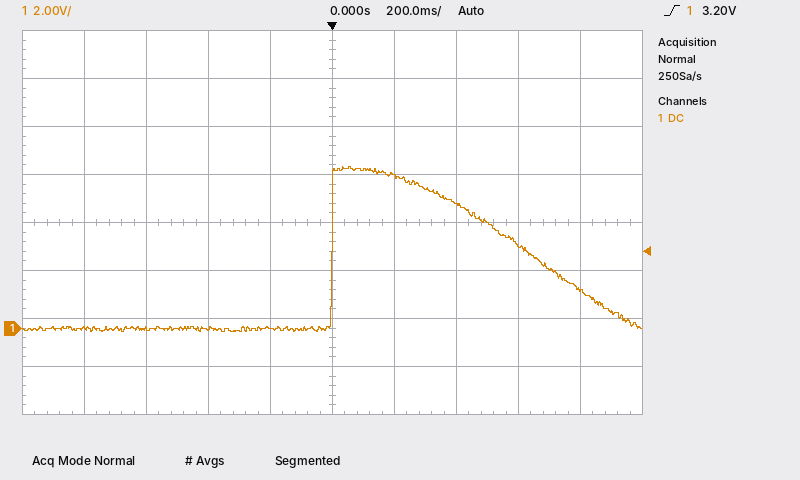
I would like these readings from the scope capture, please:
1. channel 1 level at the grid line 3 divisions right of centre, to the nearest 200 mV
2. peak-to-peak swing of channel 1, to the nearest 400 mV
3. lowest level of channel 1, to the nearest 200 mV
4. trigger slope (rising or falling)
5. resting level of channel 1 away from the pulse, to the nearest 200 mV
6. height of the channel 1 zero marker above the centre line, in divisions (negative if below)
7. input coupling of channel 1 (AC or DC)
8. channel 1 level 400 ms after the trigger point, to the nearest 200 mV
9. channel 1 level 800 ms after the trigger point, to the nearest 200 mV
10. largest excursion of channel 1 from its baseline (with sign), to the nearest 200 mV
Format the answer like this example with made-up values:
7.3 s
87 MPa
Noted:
3.4 V
6.8 V
-200 mV
rising
0.0 V
-2.2 div
DC
5.2 V
1.6 V
+6.8 V
